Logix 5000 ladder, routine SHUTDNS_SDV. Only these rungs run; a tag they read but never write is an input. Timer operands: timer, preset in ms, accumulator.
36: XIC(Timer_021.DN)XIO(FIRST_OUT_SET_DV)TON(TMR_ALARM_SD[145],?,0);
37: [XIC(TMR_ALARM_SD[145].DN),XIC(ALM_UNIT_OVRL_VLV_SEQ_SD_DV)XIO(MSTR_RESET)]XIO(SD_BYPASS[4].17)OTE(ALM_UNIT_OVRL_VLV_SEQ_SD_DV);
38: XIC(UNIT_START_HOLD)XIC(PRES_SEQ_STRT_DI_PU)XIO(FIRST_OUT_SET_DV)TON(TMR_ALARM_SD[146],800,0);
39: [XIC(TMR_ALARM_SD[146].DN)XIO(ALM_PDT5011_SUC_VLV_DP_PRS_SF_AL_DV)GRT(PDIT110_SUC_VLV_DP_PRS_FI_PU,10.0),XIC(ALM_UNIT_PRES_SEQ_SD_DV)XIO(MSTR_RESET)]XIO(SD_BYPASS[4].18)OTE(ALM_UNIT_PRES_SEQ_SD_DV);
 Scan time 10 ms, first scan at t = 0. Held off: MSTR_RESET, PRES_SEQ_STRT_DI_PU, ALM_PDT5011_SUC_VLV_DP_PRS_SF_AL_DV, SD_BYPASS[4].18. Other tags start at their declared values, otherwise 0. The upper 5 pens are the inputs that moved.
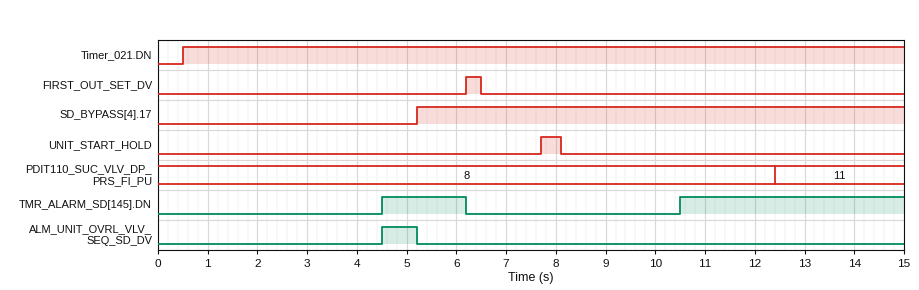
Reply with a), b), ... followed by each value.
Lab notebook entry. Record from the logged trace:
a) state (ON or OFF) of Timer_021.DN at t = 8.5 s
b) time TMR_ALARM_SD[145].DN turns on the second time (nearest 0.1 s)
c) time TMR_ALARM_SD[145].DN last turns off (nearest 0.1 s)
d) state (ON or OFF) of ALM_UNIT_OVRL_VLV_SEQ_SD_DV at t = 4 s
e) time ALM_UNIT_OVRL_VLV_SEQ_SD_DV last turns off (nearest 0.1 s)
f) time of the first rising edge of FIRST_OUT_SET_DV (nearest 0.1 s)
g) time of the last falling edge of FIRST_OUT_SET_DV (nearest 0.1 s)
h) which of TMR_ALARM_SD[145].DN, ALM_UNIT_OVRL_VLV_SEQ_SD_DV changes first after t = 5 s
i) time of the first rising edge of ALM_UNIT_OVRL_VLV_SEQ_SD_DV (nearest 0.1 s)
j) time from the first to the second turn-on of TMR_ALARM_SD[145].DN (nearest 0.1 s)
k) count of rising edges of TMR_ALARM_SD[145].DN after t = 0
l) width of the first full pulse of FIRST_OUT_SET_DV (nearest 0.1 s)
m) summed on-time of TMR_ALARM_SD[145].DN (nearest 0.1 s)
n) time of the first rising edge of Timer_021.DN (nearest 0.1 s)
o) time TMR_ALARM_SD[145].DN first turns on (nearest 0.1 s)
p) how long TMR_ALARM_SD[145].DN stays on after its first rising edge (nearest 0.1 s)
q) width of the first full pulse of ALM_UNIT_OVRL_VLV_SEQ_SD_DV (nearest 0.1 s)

a) ON
b) 10.5 s
c) 6.2 s
d) OFF
e) 5.2 s
f) 6.2 s
g) 6.5 s
h) ALM_UNIT_OVRL_VLV_SEQ_SD_DV
i) 4.5 s
j) 6.0 s
k) 2
l) 0.3 s
m) 6.2 s
n) 0.5 s
o) 4.5 s
p) 1.7 s
q) 0.7 s
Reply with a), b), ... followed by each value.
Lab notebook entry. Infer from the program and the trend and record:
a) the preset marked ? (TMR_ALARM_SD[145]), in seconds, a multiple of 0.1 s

a) 4.0 s
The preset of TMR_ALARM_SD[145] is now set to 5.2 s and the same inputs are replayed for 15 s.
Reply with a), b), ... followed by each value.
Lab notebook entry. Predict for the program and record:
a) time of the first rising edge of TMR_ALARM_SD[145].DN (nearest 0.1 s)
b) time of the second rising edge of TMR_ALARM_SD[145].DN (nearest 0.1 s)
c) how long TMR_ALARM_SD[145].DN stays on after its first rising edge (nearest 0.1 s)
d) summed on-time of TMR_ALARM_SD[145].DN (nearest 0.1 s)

a) 5.7 s
b) 11.7 s
c) 0.5 s
d) 3.8 s
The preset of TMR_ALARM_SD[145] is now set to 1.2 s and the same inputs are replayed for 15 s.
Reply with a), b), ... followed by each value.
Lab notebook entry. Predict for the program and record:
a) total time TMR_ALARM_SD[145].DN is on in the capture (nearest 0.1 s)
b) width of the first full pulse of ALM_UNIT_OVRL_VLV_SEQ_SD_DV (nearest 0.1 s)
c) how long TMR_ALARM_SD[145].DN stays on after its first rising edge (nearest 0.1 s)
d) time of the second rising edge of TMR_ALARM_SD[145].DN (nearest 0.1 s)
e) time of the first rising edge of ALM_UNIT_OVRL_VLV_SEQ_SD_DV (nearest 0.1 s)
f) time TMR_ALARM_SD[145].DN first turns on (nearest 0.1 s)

a) 11.8 s
b) 3.5 s
c) 4.5 s
d) 7.7 s
e) 1.7 s
f) 1.7 s
